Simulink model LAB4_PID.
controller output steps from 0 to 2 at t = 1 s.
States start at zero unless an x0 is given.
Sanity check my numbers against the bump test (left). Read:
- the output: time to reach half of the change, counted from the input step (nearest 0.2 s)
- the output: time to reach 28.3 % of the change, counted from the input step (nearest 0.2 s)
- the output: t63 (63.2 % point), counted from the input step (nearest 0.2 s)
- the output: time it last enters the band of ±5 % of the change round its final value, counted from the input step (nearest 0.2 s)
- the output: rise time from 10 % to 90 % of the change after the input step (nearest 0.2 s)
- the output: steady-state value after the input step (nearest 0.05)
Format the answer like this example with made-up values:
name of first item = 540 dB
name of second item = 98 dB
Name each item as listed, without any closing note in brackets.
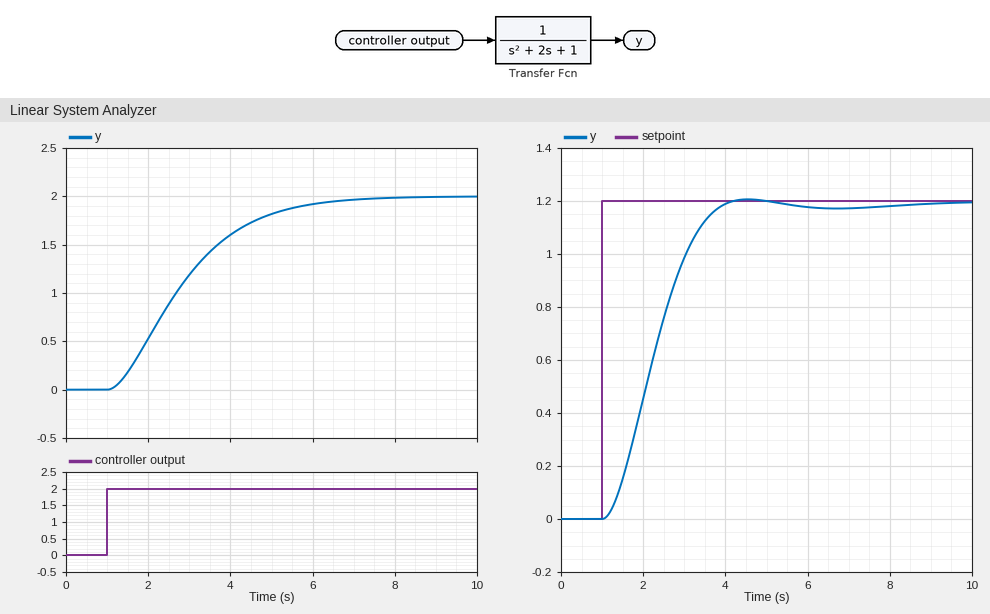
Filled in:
the output: time to reach half of the change, counted from the input step = 1.6 s
the output: time to reach 28.3 % of the change, counted from the input step = 1.0 s
the output: t63 (63.2 % point), counted from the input step = 2.2 s
the output: time it last enters the band of ±5 % of the change round its final value, counted from the input step = 4.8 s
the output: rise time from 10 % to 90 % of the change after the input step = 3.4 s
the output: steady-state value after the input step = 2.00
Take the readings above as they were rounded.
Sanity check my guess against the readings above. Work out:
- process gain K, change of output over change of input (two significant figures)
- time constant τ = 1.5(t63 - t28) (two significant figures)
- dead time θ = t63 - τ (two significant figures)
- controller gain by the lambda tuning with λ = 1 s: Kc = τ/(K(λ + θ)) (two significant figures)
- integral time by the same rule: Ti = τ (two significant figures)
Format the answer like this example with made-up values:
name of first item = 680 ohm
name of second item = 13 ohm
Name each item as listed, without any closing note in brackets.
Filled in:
process gain K, change of output over change of input = 1.0
time constant τ = 1.5(t63 - t28) = 1.8 s
dead time θ = t63 - τ = 0.40 s
controller gain by the lambda tuning with λ = 1 s: Kc = τ/(K(λ + θ)) = 1.3
integral time by the same rule: Ti = τ = 1.8 s
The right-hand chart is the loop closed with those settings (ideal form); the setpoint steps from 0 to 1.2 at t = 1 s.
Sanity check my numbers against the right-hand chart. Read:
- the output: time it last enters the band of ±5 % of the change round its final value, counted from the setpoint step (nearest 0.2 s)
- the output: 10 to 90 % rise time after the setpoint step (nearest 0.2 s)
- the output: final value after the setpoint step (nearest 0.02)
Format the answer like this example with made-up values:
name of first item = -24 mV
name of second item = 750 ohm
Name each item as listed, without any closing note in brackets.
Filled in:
the output: time it last enters the band of ±5 % of the change round its final value, counted from the setpoint step = 2.6 s
the output: 10 to 90 % rise time after the setpoint step = 1.8 s
the output: final value after the setpoint step = 1.20
